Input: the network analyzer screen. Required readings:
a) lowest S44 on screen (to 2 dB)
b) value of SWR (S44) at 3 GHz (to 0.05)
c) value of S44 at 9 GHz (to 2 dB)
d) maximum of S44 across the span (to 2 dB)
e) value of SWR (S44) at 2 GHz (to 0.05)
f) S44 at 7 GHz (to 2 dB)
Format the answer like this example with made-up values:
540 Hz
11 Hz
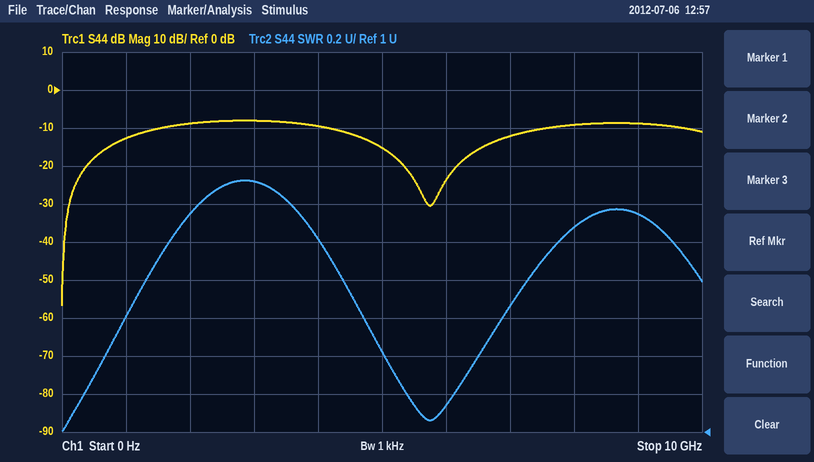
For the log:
-56 dB
2.30
-8 dB
-8 dB
2.15
-12 dB
